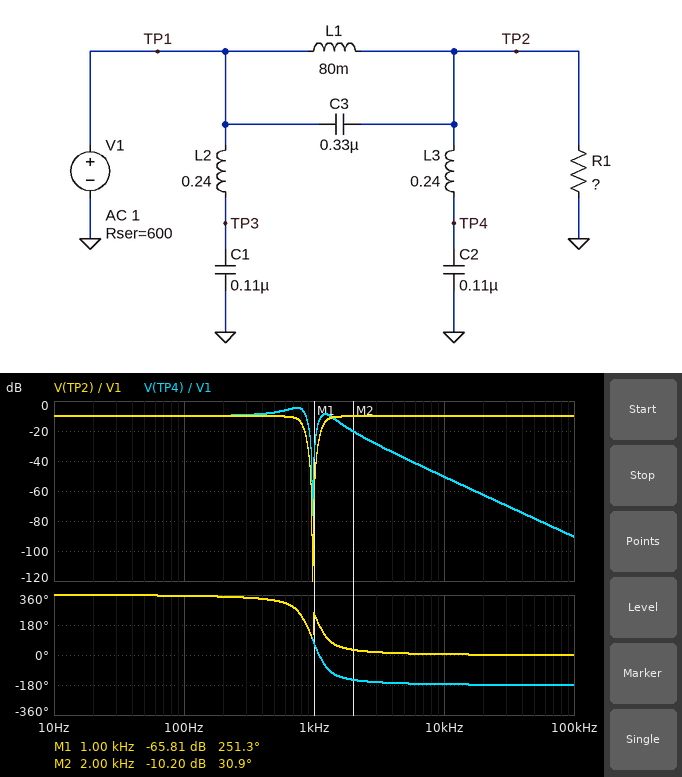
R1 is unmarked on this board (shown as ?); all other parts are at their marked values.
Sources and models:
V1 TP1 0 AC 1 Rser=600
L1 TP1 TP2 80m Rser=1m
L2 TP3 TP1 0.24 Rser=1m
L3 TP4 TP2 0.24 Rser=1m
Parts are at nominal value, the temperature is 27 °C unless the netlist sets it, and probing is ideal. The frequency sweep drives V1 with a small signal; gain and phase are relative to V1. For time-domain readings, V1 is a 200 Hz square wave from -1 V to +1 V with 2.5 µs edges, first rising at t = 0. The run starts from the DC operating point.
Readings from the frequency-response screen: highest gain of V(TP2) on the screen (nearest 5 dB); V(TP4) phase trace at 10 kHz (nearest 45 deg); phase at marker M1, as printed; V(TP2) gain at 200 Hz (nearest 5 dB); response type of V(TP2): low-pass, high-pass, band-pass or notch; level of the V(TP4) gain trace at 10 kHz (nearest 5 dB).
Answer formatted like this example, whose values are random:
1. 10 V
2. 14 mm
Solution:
1. -10 dB
2. -180 deg
3. 251.3 deg
4. -10 dB
5. notch
6. -50 dB
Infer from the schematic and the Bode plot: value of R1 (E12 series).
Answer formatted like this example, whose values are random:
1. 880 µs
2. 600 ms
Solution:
1. 270 Ω
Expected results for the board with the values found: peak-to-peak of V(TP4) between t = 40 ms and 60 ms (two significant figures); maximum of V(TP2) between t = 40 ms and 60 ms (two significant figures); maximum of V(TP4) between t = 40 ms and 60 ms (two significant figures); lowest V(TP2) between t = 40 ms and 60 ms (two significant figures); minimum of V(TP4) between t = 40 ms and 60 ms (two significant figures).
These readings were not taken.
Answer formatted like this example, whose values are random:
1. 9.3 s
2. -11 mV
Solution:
1. 910 mV
2. 440 mV
3. 450 mV
4. -440 mV
5. -450 mV
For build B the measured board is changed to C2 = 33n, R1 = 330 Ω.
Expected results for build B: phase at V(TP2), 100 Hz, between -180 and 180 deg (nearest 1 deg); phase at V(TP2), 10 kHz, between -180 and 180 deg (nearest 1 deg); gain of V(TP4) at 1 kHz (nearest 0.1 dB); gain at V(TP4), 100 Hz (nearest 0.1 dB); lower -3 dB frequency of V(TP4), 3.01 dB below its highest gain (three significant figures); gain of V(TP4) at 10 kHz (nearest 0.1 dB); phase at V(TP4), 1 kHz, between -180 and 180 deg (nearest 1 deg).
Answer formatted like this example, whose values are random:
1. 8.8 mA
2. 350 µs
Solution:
1. -4 deg
2. 5 deg
3. -47.8 dB
4. -9.0 dB
5. 1.72 kHz
6. -38.6 dB
7. 167 deg
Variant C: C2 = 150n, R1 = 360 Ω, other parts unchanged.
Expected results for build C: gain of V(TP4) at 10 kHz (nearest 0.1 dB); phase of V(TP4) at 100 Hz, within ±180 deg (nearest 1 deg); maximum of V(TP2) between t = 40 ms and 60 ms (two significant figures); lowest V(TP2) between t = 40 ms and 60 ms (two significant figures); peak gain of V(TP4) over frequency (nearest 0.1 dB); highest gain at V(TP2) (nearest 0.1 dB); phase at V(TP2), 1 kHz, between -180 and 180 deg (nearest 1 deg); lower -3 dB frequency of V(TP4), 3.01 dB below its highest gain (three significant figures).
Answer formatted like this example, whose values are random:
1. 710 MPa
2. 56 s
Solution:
1. -51.5 dB
2. -5 deg
3. 530 mV
4. -530 mV
5. 2.2 dB
6. -8.5 dB
7. -148 deg
8. 654 Hz
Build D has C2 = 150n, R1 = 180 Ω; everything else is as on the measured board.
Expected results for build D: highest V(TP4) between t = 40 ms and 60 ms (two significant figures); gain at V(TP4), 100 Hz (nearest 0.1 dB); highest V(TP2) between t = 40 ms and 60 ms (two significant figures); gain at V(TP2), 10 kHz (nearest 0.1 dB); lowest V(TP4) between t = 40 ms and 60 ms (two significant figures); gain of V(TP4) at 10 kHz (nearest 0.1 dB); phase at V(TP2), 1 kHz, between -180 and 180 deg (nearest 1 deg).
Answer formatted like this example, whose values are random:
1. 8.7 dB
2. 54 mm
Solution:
1. 380 mV
2. -12.6 dB
3. 320 mV
4. -12.7 dB
5. -380 mV
6. -55.7 dB
7. -165 deg
